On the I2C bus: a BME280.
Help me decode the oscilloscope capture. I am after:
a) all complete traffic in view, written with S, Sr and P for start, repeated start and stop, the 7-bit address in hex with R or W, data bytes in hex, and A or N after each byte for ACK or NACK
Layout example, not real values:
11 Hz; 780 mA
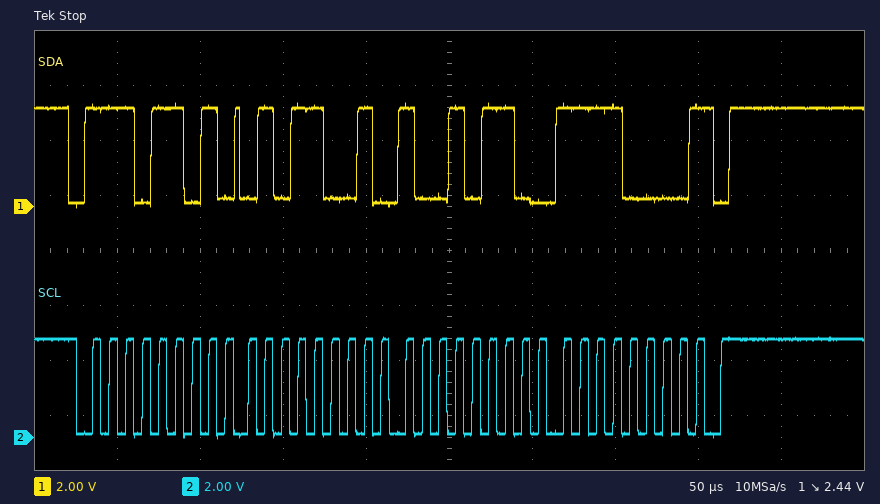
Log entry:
S 76R A 59 A 96 A F0 N P
